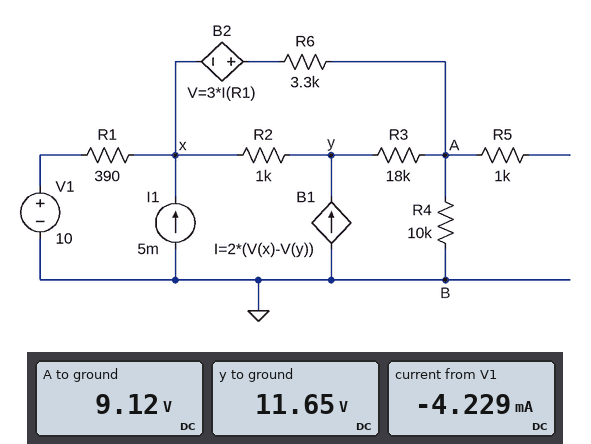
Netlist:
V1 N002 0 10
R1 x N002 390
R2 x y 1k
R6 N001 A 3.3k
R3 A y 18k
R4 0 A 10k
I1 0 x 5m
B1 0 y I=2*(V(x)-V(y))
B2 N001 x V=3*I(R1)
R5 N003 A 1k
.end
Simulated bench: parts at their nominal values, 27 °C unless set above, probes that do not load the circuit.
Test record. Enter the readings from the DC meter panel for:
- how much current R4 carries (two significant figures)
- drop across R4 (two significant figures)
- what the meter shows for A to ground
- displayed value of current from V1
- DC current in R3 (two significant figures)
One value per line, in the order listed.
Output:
910 µA
9.1 V
9.12 V
-4.229 mA
140 µA
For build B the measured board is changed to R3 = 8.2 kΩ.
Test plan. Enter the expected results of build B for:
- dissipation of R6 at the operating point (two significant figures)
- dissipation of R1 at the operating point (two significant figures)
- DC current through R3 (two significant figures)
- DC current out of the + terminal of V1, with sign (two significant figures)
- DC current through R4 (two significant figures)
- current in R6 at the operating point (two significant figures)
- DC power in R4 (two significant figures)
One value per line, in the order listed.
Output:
1.5 mW
7.3 mW
270 µA
-4.3 mA
950 µA
680 µA
9.0 mW
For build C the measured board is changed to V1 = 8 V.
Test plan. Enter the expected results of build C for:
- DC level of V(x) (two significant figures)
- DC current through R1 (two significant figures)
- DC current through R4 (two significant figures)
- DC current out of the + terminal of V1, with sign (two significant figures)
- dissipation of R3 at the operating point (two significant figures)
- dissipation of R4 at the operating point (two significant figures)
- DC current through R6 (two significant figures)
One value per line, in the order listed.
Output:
9.7 V
4.4 mA
760 µA
-4.4 mA
250 µW
5.8 mW
640 µA
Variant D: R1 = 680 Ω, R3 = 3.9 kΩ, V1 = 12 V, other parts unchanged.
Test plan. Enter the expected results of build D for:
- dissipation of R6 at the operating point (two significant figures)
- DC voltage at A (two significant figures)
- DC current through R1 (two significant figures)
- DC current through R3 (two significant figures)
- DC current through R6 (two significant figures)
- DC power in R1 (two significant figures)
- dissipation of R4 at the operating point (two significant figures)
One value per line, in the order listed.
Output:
1.6 mW
13 V
4.3 mA
580 µA
690 µA
13 mW
16 mW
